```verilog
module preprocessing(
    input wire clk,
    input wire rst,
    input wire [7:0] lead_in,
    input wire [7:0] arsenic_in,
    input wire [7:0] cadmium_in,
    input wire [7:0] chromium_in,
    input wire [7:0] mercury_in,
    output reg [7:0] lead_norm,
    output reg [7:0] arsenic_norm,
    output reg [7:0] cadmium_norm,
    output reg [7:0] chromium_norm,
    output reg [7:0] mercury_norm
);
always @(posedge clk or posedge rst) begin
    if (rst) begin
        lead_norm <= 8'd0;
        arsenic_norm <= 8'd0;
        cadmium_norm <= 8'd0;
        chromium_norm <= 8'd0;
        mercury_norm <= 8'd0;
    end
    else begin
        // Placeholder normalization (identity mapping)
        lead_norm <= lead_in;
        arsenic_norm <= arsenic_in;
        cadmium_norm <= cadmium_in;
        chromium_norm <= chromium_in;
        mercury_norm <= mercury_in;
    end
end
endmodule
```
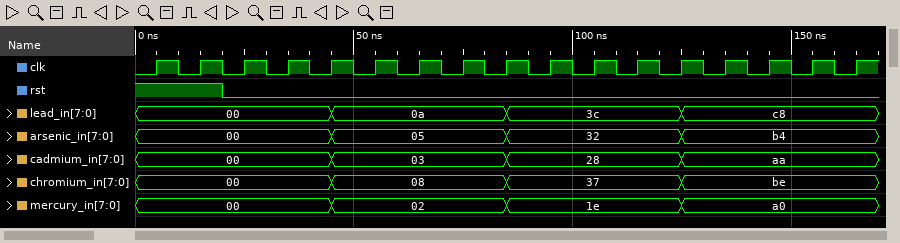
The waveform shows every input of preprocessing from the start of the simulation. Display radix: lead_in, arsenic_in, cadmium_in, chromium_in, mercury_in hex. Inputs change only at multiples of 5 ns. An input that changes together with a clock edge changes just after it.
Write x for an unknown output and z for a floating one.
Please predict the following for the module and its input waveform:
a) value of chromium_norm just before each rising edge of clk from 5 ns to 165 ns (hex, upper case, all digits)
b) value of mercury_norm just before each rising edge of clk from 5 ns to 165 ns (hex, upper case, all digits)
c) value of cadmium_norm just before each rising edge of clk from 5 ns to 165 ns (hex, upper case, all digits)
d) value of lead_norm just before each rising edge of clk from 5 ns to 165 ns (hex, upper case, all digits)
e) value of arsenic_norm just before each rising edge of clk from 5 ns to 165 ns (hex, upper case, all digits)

00, 00, 00, 00, 00, 00, 08, 08, 08, 08, 37, 37, 37, 37, BE, BE, BE
00, 00, 00, 00, 00, 00, 02, 02, 02, 02, 1E, 1E, 1E, 1E, A0, A0, A0
00, 00, 00, 00, 00, 00, 03, 03, 03, 03, 28, 28, 28, 28, AA, AA, AA
00, 00, 00, 00, 00, 00, 0A, 0A, 0A, 0A, 3C, 3C, 3C, 3C, C8, C8, C8
00, 00, 00, 00, 00, 00, 05, 05, 05, 05, 32, 32, 32, 32, B4, B4, B4
